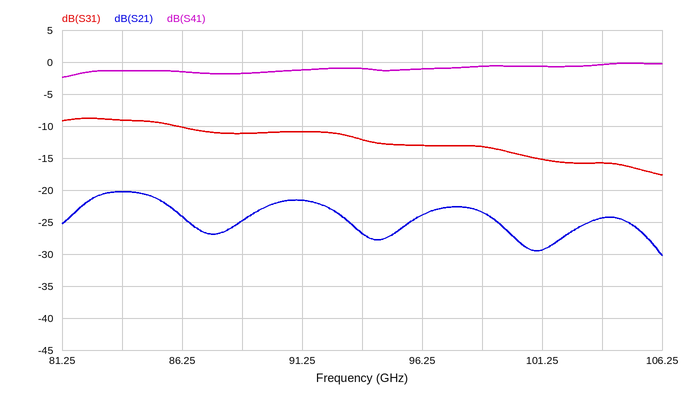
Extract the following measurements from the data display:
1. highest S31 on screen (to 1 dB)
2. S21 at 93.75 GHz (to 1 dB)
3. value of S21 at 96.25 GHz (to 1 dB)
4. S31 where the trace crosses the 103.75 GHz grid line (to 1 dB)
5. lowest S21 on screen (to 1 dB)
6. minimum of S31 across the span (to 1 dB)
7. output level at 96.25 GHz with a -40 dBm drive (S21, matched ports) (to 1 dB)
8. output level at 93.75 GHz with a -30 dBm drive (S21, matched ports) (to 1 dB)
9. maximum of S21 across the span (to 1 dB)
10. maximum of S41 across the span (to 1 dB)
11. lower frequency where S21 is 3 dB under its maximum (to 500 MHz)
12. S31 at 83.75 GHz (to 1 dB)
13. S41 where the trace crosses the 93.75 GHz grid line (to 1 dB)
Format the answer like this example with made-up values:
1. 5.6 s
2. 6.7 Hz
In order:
1. -9 dB
2. -27 dB
3. -24 dB
4. -16 dB
5. -30 dB
6. -18 dB
7. -64 dBm
8. -57 dBm
9. -20 dB
10. 0 dB
11. 82.0 GHz
12. -9 dB
13. -1 dB
